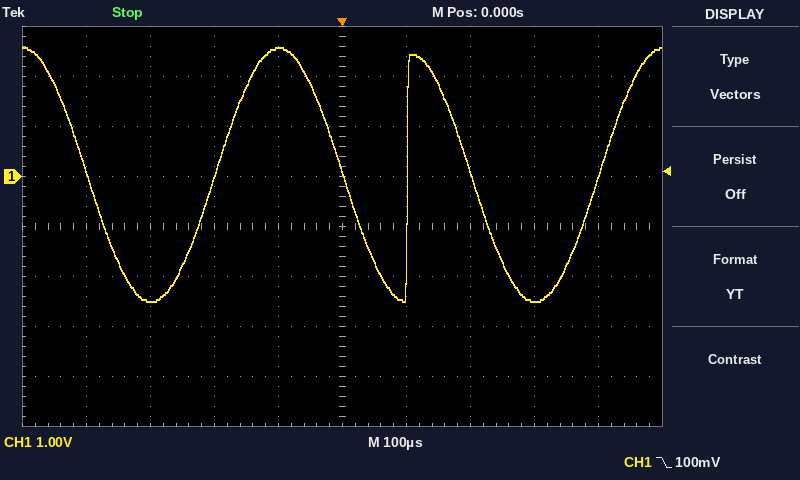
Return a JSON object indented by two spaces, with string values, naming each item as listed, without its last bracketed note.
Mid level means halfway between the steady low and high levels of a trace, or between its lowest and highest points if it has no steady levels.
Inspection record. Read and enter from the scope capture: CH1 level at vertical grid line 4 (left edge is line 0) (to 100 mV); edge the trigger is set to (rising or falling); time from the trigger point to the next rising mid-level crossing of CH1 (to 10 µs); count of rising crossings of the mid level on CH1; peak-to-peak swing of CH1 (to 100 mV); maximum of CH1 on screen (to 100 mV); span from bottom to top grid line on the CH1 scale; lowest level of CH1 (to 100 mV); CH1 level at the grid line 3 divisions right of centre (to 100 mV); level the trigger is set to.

{
  "CH1 level at vertical grid line 4 (left edge is line 0)": "2.6 V",
  "edge the trigger is set to": "falling",
  "time from the trigger point to the next rising mid-level crossing of CH1": "100 µs",
  "count of rising crossings of the mid level on CH1": "3",
  "peak-to-peak swing of CH1": "5.1 V",
  "maximum of CH1 on screen": "2.6 V",
  "span from bottom to top grid line on the CH1 scale": "8 V",
  "lowest level of CH1": "-2.5 V",
  "CH1 level at the grid line 3 divisions right of centre": "-2.5 V",
  "level the trigger is set to": "100 mV"
}
